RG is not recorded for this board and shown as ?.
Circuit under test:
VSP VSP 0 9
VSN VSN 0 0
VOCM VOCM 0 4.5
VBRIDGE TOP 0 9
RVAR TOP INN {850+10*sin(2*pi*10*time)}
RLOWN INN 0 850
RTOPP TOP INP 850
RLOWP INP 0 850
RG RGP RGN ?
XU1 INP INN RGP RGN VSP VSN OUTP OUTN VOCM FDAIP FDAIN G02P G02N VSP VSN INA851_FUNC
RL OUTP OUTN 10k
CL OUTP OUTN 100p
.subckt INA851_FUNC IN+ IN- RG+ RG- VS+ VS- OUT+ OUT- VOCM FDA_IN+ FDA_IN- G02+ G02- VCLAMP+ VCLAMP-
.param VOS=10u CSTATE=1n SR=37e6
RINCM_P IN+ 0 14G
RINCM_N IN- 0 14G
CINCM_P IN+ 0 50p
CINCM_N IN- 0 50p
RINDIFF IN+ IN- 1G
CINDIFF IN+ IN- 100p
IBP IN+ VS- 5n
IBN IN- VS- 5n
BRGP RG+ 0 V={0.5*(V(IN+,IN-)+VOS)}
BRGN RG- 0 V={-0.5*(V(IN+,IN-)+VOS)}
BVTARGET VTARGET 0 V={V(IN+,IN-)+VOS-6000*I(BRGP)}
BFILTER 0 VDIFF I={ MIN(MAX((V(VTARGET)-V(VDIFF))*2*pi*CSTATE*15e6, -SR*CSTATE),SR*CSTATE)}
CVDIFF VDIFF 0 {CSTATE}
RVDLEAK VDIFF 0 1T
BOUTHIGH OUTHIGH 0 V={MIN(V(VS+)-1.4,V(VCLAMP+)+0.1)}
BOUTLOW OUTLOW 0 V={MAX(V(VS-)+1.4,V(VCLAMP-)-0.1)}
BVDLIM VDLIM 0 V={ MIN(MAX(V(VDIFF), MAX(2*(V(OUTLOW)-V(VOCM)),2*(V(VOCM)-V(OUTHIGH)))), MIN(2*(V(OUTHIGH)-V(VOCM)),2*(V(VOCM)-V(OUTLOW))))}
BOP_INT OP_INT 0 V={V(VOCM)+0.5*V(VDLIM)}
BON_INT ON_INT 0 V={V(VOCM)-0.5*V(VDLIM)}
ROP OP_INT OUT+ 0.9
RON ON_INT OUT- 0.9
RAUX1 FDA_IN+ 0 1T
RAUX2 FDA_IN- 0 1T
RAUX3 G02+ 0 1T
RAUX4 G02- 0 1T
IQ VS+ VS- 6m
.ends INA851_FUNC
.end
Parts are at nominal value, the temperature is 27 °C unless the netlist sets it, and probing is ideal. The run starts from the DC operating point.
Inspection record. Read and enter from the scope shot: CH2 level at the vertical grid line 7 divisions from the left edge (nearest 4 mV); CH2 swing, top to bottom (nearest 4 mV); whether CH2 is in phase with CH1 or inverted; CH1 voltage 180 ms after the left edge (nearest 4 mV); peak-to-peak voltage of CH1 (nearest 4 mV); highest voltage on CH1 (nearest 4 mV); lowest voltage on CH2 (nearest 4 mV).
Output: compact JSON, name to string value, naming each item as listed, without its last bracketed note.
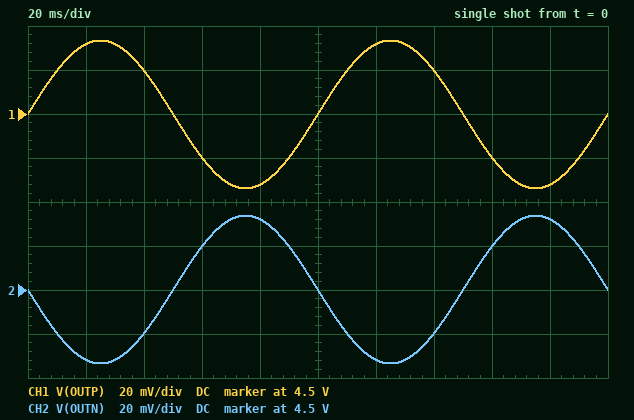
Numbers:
{"CH2 level at the vertical grid line 7 divisions from the left edge": "4.480 V", "CH2 swing, top to bottom": "68 mV", "whether CH2 is in phase with CH1 or inverted": "inverted", "CH1 voltage 180 ms after the left edge": "4.468 V", "peak-to-peak voltage of CH1": "68 mV", "highest voltage on CH1": "4.532 V", "lowest voltage on CH2": "4.468 V"}
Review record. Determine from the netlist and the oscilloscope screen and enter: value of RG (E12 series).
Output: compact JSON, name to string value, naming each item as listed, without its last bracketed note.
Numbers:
{"value of RG": "3.9 kΩ"}
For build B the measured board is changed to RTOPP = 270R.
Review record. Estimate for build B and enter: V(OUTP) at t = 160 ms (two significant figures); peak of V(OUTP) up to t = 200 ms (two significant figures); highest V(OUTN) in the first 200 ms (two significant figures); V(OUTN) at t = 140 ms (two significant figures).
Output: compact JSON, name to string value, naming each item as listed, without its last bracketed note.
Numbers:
{"V(OUTP) at t = 160 ms": "7.4 V", "peak of V(OUTP) up to t = 200 ms": "7.5 V", "highest V(OUTN) in the first 200 ms": "1.6 V", "V(OUTN) at t = 140 ms": "1.5 V"}
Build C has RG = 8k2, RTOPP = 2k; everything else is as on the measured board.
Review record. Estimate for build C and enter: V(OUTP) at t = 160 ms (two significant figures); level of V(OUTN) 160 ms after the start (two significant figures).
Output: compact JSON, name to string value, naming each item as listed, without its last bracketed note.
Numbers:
{"V(OUTP) at t = 160 ms": "2.9 V", "level of V(OUTN) 160 ms after the start": "6.1 V"}
